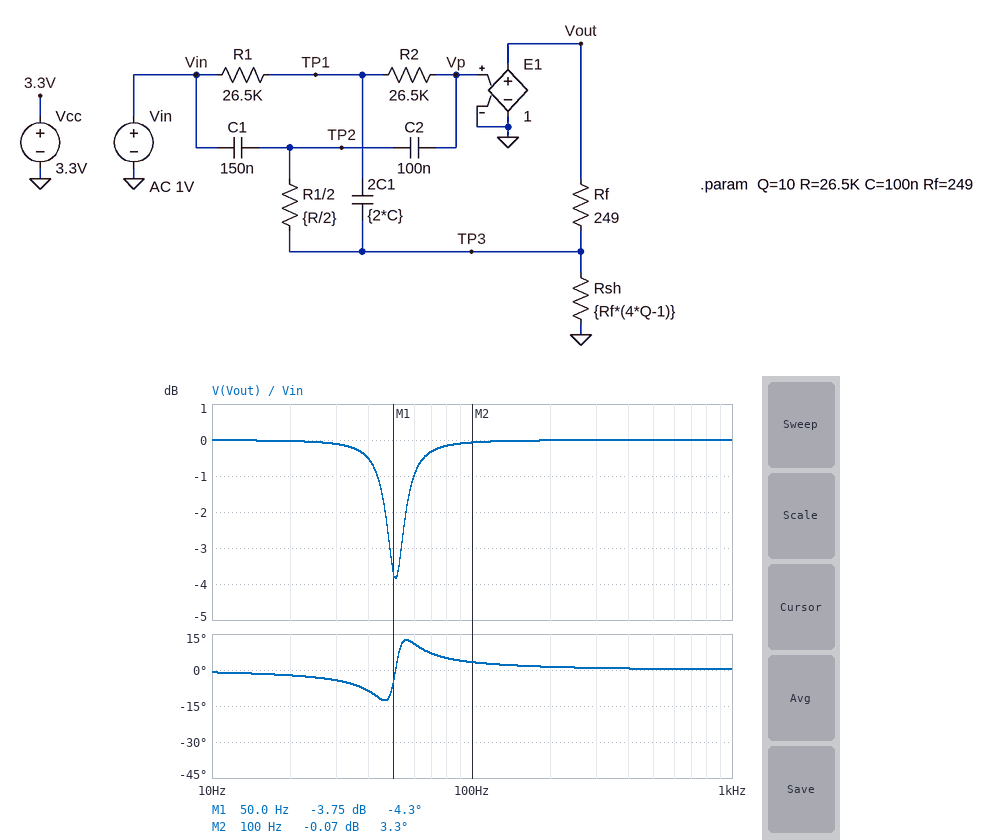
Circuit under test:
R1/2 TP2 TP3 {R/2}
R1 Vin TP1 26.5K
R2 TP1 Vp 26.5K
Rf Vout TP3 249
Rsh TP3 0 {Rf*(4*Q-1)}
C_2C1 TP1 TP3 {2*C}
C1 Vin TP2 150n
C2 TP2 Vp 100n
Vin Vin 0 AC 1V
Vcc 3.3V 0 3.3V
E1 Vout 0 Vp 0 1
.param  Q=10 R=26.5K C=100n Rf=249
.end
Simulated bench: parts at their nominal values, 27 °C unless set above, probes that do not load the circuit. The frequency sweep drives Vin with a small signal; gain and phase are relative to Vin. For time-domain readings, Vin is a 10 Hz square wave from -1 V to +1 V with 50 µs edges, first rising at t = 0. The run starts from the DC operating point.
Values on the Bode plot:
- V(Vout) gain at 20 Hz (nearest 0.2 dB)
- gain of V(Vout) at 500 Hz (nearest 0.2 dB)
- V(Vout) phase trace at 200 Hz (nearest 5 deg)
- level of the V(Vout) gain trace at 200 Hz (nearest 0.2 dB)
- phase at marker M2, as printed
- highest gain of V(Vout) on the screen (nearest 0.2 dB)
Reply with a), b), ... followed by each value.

a) 0 dB
b) 0 dB
c) 0 deg
d) 0 dB
e) 3.3 deg
f) 0 dB
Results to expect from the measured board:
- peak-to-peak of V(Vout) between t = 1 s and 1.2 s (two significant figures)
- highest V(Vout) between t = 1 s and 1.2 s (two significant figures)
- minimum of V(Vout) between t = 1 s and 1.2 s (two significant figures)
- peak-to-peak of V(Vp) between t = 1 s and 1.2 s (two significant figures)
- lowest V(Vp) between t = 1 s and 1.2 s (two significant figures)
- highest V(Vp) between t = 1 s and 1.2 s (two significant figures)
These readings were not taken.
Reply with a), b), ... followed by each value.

a) 2.2 V
b) 1.1 V
c) -1.1 V
d) 2.2 V
e) -1.1 V
f) 1.1 V
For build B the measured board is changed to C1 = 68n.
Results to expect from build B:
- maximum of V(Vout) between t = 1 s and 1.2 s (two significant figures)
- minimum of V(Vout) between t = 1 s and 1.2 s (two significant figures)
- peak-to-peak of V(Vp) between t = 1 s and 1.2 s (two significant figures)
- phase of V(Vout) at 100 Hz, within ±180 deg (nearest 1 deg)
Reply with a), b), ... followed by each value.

a) 1.3 V
b) -1.3 V
c) 2.6 V
d) 8 deg
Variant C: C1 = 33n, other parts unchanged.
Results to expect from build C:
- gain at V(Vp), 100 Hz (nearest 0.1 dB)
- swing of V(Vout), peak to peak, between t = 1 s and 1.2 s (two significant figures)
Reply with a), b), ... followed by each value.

a) 1.2 dB
b) 3.7 V
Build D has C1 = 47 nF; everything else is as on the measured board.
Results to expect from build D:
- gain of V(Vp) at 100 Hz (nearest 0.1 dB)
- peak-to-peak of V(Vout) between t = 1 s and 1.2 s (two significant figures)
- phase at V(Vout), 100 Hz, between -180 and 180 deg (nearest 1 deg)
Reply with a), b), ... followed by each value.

a) 0.1 dB
b) 2.3 V
c) 16 deg
